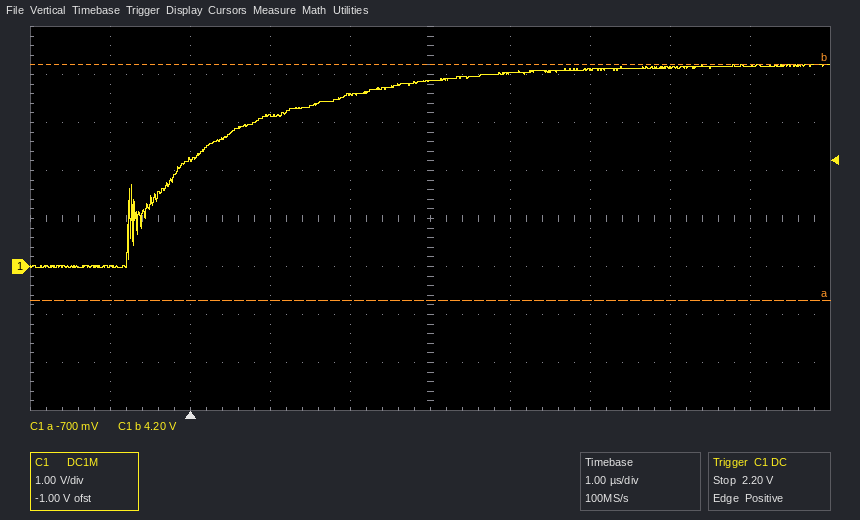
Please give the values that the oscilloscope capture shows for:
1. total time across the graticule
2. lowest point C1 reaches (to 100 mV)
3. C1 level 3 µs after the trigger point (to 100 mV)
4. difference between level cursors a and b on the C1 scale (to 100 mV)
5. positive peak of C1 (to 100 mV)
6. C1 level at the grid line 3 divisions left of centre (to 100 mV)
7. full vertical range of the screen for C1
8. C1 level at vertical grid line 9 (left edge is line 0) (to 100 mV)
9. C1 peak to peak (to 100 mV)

10 µs
0.0 V
3.9 V
4.9 V
4.2 V
2.2 V
8 V
4.2 V
4.2 V
